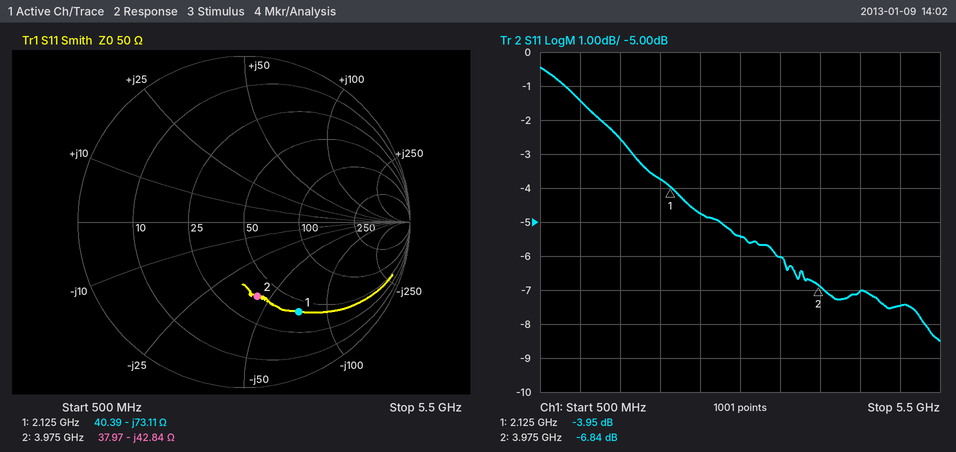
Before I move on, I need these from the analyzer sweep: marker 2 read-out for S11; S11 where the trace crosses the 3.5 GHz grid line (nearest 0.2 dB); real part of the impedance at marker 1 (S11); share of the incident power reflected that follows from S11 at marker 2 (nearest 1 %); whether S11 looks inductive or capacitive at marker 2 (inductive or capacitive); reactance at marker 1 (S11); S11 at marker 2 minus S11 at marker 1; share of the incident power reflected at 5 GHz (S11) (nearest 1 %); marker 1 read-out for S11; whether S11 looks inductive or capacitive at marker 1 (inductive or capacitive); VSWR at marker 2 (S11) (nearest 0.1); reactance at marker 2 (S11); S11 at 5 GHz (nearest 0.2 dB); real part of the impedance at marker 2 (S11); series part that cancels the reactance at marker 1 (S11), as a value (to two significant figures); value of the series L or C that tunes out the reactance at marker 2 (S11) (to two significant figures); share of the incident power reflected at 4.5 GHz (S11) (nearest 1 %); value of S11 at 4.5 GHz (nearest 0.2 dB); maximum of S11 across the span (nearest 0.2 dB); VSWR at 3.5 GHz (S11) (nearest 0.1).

-6.84 dB
-6.0 dB
40.39 Ω
21 %
capacitive
-73.11 Ω
-2.89 dB
18 %
-3.95 dB
capacitive
2.7
-42.84 Ω
-7.4 dB
37.97 Ω
5.5 nH
1.7 nH
20 %
-7.0 dB
-0.4 dB
3.0
